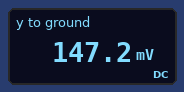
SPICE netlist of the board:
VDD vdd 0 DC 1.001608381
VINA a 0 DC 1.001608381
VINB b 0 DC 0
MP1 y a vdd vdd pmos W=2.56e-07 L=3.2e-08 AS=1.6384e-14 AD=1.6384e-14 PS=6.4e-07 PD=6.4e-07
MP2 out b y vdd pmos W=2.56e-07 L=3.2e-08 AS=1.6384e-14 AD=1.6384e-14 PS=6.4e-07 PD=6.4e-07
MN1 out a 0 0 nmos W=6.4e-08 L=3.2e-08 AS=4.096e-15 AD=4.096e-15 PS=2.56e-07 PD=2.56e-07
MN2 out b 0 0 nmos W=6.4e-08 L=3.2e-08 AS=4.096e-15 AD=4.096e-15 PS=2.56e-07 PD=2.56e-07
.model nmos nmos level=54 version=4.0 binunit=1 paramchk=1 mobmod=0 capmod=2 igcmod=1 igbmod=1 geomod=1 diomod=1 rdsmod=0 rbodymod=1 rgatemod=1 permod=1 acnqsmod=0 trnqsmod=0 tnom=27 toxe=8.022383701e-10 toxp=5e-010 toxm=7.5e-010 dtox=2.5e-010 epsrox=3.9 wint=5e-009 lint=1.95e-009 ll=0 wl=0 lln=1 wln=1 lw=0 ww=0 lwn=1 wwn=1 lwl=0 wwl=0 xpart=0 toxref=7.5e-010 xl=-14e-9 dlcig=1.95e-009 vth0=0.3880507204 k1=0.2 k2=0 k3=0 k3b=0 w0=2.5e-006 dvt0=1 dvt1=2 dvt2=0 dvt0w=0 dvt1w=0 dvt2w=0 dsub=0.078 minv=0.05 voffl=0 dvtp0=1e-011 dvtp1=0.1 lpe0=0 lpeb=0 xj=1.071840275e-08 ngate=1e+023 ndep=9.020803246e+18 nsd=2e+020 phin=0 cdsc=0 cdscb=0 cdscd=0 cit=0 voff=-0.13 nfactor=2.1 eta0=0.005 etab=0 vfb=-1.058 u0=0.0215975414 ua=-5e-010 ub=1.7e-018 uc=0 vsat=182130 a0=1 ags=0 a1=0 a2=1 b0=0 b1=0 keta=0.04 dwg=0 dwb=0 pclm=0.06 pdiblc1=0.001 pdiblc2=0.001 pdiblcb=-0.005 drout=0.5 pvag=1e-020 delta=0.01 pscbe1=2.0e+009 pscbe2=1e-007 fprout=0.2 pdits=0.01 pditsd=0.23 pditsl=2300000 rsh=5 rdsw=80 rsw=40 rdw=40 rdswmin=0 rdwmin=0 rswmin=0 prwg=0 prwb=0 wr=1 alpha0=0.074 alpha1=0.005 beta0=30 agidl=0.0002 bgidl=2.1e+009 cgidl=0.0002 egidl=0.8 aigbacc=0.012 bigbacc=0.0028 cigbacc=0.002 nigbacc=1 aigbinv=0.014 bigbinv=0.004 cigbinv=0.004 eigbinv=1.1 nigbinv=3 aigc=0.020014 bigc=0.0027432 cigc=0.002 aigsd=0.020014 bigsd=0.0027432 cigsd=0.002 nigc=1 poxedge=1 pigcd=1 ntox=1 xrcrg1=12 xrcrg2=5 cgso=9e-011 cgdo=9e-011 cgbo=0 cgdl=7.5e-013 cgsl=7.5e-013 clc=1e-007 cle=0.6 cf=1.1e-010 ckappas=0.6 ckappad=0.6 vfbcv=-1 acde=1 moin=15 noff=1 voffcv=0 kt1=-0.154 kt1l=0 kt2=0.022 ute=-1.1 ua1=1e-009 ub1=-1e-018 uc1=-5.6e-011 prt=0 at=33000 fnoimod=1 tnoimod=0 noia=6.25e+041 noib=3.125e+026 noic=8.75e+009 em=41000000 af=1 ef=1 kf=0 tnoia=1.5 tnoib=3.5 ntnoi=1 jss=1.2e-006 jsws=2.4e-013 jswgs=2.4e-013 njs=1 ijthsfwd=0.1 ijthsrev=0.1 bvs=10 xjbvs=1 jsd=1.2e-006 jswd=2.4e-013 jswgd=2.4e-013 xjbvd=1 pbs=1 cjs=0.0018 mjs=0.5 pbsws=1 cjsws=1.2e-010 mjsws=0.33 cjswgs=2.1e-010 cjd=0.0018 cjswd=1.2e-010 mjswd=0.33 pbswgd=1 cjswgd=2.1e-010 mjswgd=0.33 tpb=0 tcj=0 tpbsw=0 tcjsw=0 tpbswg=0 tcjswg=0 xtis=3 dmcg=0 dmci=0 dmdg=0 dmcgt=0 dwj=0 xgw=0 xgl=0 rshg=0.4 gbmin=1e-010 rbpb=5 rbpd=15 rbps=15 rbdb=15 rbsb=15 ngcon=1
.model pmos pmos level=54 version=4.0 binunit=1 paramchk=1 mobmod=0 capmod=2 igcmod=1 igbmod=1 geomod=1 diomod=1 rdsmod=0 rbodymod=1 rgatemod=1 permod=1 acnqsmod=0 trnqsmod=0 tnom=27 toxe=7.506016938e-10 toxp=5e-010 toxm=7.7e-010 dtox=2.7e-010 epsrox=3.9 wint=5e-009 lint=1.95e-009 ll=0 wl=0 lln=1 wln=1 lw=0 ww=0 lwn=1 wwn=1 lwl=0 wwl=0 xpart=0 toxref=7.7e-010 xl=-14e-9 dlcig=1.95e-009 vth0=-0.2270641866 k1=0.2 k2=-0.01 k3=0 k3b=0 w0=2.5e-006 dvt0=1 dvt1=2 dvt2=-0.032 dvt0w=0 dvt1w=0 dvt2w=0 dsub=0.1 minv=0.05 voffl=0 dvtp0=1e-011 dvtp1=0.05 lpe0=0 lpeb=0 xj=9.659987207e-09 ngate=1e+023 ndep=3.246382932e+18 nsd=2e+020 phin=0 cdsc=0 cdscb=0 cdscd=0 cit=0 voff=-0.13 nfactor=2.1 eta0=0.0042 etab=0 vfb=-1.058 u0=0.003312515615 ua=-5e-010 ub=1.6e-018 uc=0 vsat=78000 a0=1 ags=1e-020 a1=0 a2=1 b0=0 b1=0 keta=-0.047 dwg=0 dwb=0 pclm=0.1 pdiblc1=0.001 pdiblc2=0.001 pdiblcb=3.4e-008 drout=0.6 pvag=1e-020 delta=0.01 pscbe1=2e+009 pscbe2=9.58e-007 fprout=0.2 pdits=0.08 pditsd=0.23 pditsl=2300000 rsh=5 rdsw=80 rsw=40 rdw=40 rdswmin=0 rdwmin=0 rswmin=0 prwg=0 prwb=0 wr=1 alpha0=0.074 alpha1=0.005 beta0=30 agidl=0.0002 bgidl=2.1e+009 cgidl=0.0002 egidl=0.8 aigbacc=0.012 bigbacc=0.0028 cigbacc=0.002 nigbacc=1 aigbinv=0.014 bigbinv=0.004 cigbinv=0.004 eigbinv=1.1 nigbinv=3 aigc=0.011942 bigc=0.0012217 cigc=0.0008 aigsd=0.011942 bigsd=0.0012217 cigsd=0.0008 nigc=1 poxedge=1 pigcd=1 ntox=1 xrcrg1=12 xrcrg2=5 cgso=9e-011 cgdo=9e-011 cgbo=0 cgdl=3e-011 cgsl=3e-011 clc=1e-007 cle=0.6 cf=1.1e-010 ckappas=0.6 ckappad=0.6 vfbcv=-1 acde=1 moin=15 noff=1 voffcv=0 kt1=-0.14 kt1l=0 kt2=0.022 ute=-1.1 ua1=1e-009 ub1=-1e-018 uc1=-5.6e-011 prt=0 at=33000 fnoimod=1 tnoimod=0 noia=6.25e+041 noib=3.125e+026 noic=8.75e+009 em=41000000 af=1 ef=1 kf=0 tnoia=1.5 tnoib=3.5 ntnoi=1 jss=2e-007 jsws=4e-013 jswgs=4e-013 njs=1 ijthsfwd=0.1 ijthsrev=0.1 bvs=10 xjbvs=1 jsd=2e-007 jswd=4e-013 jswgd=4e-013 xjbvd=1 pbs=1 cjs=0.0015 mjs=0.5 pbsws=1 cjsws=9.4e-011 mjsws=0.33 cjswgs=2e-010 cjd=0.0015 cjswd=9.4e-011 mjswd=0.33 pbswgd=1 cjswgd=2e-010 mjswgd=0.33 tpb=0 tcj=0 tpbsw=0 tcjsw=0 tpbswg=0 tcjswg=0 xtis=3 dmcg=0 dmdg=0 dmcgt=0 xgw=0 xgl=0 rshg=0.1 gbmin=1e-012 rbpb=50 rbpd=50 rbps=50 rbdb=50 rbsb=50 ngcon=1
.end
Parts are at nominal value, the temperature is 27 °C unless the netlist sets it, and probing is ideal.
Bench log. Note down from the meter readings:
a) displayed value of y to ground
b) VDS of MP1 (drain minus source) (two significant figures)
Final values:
147.2 mV
-850 mV
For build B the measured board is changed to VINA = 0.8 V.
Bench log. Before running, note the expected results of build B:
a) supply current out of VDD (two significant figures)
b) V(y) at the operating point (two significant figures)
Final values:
9.1 µA
310 mV
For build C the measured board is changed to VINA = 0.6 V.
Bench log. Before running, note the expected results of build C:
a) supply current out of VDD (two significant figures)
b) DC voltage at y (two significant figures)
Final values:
43 µA
720 mV
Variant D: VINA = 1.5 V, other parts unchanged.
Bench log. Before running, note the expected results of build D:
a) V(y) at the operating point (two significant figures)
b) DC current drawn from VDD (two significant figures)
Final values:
200 mV
790 nA
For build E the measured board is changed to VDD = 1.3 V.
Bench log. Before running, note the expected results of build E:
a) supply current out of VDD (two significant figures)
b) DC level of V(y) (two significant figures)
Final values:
36 µA
450 mV
